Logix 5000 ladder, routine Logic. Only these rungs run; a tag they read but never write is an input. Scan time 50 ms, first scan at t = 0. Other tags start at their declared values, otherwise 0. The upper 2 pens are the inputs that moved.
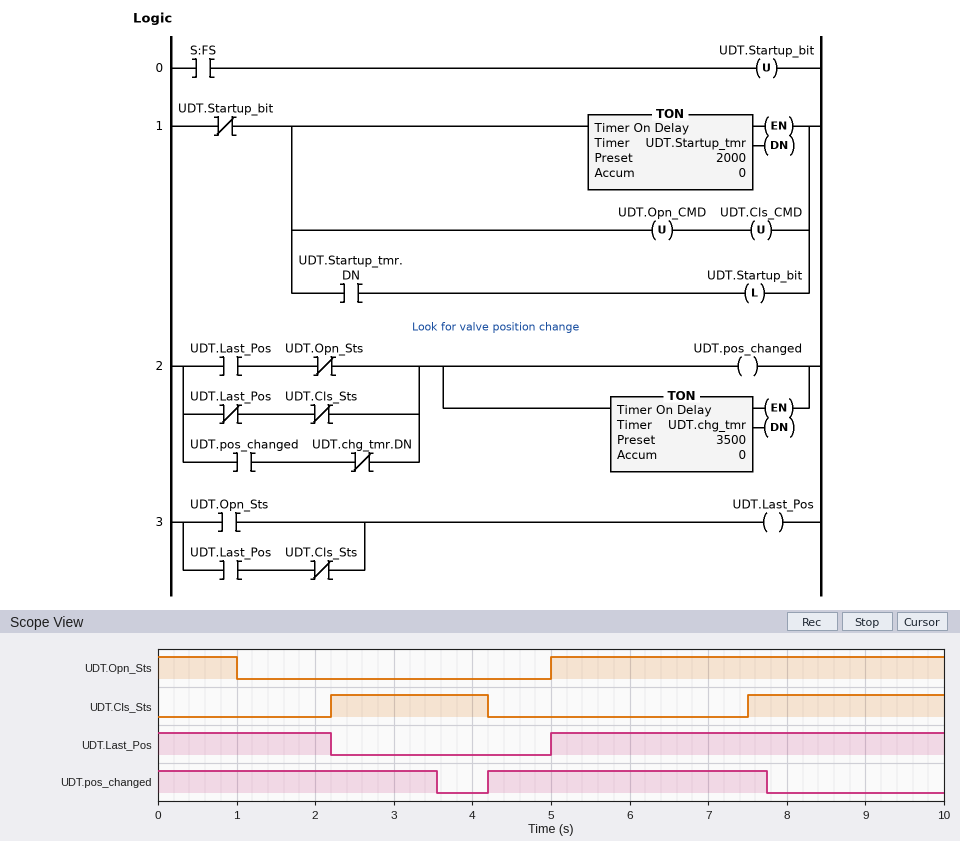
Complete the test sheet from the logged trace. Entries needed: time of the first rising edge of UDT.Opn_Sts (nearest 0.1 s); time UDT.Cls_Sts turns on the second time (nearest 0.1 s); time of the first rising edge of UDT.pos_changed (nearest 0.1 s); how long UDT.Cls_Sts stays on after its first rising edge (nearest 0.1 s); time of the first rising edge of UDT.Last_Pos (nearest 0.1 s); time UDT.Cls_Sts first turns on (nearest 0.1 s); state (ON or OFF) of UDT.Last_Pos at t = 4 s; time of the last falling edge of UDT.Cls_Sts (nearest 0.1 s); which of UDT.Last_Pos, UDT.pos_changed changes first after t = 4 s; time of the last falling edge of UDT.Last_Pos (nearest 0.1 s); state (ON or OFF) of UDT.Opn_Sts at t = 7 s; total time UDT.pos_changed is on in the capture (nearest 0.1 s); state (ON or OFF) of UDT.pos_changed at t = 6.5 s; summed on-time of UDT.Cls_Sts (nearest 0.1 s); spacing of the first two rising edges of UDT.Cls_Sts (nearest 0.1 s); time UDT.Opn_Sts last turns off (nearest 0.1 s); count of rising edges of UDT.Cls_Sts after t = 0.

5.0 s
7.5 s
4.2 s
2.0 s
5.0 s
2.2 s
OFF
4.2 s
UDT.pos_changed
2.2 s
ON
7.1 s
ON
4.5 s
5.3 s
1.0 s
2
